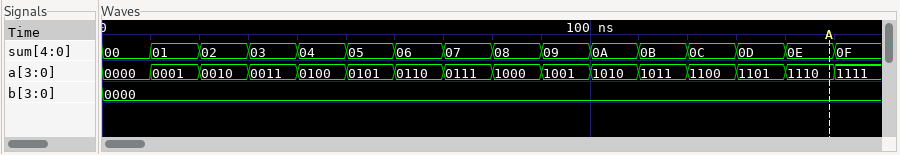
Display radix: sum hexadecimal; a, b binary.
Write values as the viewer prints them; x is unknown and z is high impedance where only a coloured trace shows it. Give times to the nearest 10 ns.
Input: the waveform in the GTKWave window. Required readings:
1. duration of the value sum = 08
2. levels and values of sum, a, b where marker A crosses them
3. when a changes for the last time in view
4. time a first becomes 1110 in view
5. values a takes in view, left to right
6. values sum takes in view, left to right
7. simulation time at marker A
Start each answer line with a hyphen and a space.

- 10 ns
- sum=0E, a=1110, b=0000
- 150 ns
- 140 ns
- 0000, 0001, 0010, 0011, 0100, 0101, 0110, 0111, 1000, 1001, 1010, 1011, 1100, 1101, 1110, 1111
- 00, 01, 02, 03, 04, 05, 06, 07, 08, 09, 0A, 0B, 0C, 0D, 0E, 0F
- 150 ns
